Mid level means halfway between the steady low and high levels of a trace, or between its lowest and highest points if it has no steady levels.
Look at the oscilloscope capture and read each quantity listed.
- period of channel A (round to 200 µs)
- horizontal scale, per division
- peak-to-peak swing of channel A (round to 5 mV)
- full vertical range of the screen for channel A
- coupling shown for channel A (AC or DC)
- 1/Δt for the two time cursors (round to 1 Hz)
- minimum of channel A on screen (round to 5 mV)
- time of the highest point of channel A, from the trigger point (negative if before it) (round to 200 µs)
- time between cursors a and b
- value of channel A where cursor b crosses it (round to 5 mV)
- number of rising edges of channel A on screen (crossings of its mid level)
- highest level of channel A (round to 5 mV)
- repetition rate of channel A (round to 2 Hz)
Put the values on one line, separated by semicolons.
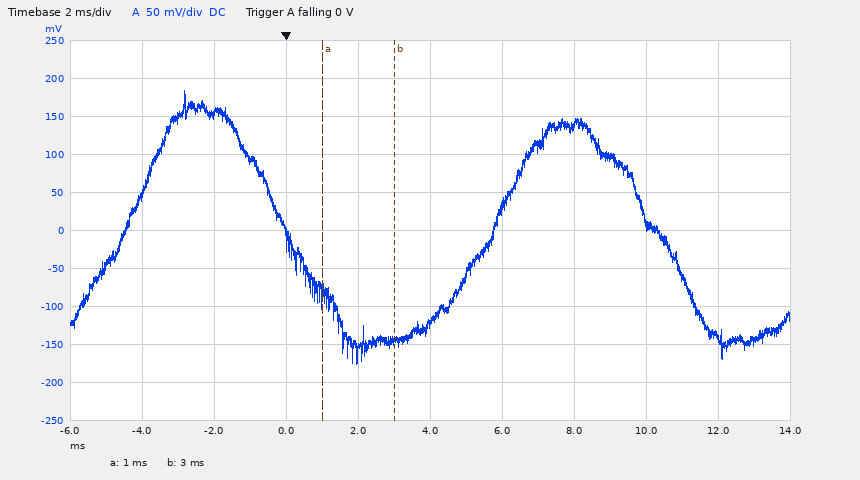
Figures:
10.2 ms; 2 ms; 360 mV; 500 mV; DC; 500 Hz; -175 mV; -2.8 ms; 2.0 ms; -145 mV; 2; 185 mV; 98 Hz
